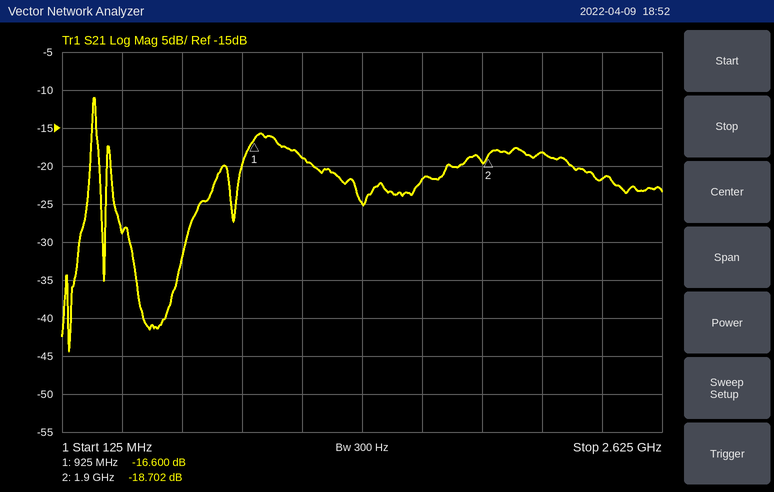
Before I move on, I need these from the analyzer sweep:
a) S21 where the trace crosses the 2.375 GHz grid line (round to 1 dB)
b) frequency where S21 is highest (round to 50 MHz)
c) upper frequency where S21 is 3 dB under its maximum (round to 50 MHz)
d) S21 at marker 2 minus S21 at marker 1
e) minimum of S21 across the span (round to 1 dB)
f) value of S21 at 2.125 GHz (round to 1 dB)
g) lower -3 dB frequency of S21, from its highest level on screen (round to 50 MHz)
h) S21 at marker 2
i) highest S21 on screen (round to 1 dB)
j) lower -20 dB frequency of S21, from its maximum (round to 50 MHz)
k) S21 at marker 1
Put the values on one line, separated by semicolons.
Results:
-22 dB; 250 MHz; 250 MHz; -2.102 dB; -44 dB; -18 dB; 250 MHz; -18.702 dB; -11 dB; 200 MHz; -16.600 dB
